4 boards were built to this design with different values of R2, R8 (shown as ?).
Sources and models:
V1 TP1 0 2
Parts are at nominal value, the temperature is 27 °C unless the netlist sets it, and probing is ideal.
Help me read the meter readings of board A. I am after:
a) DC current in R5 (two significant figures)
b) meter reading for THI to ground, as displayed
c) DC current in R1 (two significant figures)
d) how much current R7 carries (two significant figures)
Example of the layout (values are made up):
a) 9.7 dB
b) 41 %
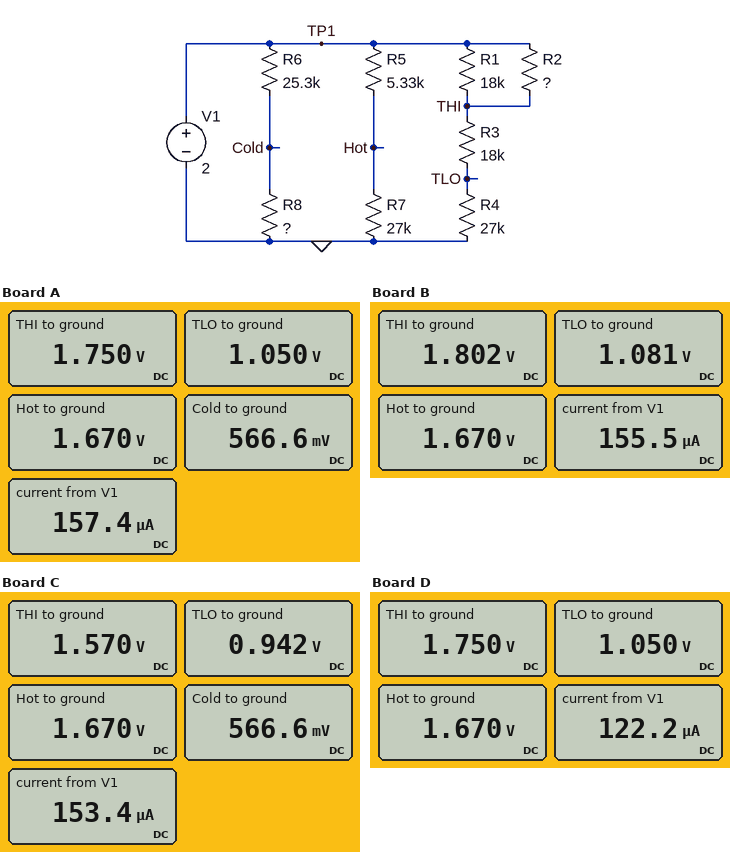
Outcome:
a) 62 µA
b) 1.750 V
c) 14 µA
d) 62 µA
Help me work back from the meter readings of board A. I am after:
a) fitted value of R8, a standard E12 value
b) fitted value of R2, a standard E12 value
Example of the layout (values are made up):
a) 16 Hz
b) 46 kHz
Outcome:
a) 10 kΩ
b) 10 kΩ
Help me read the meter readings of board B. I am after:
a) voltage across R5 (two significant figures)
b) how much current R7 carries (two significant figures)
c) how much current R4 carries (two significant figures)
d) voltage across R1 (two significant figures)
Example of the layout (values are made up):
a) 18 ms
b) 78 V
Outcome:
a) 330 mV
b) 62 µA
c) 40 µA
d) 200 mV
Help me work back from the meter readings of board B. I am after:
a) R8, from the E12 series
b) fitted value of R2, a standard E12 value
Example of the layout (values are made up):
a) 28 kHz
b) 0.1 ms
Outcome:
a) 12 kΩ
b) 6.8 kΩ
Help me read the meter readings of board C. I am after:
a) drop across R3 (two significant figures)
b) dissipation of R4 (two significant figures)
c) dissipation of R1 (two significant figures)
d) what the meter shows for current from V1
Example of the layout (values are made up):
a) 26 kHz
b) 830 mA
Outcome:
a) 630 mV
b) 33 µW
c) 10 µW
d) 153.4 µA
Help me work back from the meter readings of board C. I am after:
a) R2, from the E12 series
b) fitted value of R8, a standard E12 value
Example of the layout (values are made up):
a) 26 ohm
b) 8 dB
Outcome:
a) 39 kΩ
b) 10 kΩ
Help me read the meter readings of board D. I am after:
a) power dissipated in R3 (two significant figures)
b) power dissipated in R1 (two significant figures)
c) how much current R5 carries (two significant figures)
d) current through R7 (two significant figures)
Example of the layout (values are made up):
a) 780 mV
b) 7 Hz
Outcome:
a) 27 µW
b) 3.5 µW
c) 62 µA
d) 62 µA
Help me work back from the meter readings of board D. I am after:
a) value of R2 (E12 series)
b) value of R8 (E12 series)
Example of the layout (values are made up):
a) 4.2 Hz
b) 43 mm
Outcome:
a) 10 kΩ
b) 68 kΩ
